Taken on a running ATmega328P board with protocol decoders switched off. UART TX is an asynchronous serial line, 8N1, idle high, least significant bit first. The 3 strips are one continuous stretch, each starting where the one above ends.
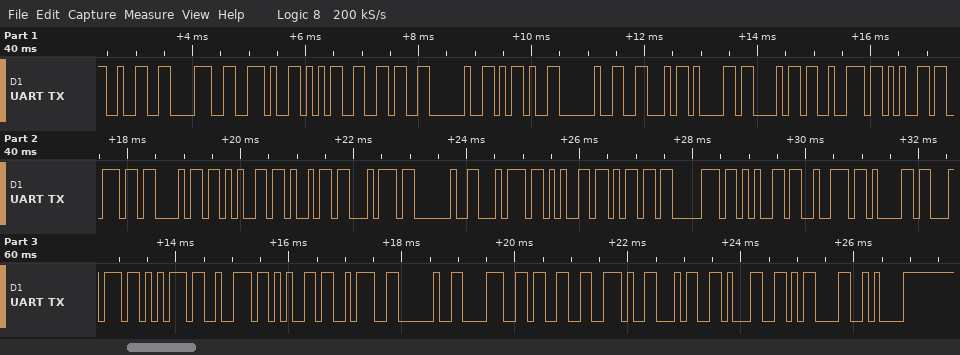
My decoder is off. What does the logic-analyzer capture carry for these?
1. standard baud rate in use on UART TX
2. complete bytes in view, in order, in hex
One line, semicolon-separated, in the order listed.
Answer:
9600 baud; 32 38 2E 35 36 20 2D 20 46 61 68 72 65 6E 68 65 69 74 20 74 65 6D 70 65 72 61 74 75 72 65 3A 20 38 33 2E 34 31 0D 0A
